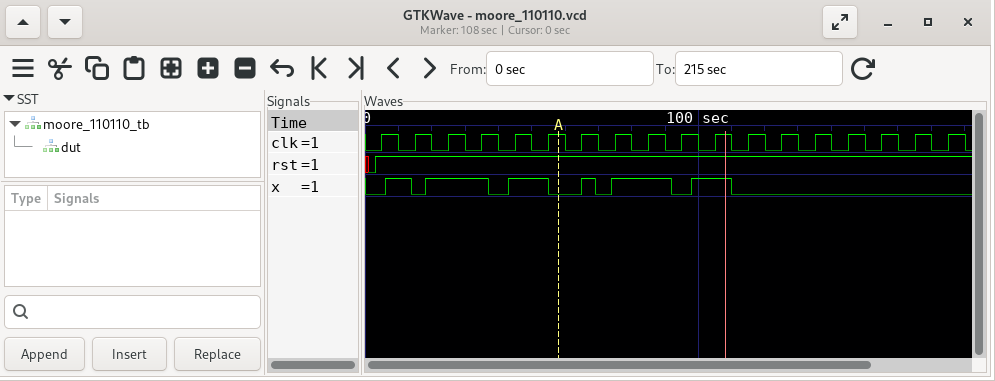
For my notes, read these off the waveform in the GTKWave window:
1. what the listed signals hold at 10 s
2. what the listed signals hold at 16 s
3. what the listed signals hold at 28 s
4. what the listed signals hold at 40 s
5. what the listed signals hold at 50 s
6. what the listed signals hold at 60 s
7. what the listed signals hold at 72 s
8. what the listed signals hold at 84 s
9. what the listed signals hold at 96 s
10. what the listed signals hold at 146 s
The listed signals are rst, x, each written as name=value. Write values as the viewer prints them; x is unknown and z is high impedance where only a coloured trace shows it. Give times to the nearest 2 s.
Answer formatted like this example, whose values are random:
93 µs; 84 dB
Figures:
rst=1, x=1; rst=1, x=0; rst=1, x=1; rst=1, x=0; rst=1, x=1; rst=1, x=0; rst=1, x=0; rst=1, x=1; rst=1, x=0; rst=1, x=0
